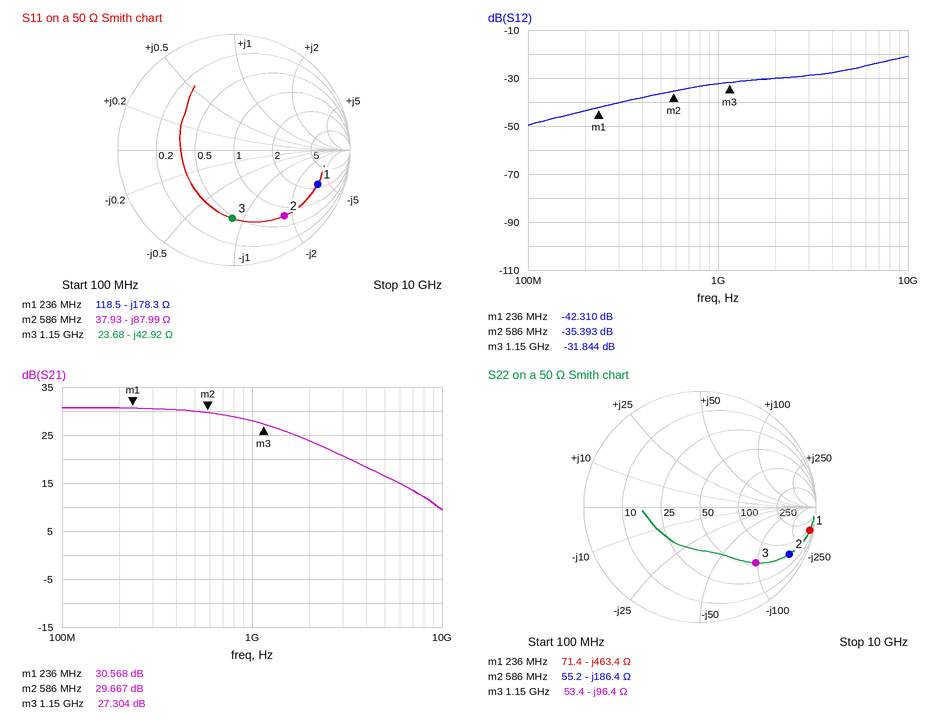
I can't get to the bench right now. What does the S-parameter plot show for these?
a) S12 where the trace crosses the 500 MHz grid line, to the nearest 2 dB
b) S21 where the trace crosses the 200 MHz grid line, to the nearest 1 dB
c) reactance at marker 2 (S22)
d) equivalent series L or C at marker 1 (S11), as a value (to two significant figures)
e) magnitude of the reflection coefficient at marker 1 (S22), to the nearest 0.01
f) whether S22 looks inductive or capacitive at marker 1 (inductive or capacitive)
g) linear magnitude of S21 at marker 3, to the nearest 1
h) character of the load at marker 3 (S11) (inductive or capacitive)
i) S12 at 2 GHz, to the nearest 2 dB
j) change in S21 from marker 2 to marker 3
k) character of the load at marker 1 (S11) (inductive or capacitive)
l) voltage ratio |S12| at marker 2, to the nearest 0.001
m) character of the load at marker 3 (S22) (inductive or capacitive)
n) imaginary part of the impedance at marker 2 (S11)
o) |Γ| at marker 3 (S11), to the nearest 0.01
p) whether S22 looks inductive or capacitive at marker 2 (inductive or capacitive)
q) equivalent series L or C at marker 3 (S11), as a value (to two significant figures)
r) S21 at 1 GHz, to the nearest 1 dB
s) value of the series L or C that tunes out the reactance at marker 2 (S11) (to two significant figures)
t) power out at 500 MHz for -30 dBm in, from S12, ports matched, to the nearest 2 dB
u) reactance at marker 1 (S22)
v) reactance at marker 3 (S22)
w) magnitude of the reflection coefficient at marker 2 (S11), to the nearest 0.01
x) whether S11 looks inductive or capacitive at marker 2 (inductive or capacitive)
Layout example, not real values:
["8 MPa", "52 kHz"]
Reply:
["-36 dB", "31 dB", "-186.4 Ω", "3.8 pF", "0.97", "capacitive", "23", "capacitive", "-30 dB", "-2.363 dB", "capacitive", "0.017", "capacitive", "-87.99 Ω", "0.59", "capacitive", "3.2 pF", "28 dB", "24 nH", "-66 dBm", "-463.4 Ω", "-96.4 Ω", "0.71", "capacitive"]
